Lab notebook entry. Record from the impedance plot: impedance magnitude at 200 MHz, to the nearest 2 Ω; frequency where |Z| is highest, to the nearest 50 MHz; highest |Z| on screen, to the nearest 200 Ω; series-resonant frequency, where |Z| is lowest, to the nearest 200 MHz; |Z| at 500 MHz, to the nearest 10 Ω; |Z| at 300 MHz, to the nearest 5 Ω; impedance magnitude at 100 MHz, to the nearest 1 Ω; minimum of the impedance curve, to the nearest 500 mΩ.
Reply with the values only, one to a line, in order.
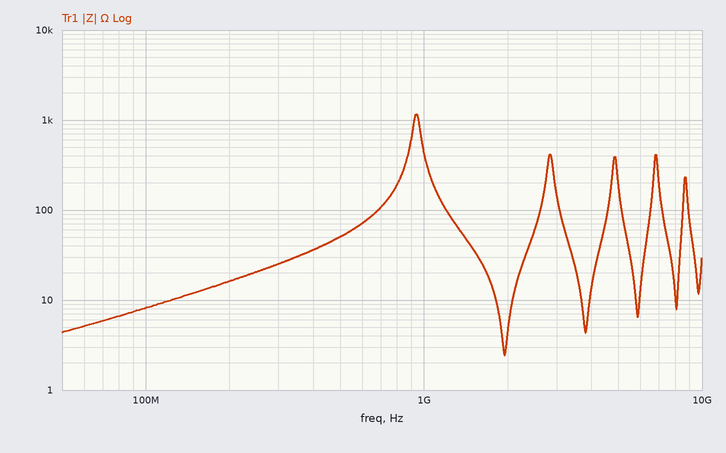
16 Ω
950 MHz
1.2 kΩ
2.0 GHz
50 Ω
25 Ω
8 Ω
2.5 Ω
